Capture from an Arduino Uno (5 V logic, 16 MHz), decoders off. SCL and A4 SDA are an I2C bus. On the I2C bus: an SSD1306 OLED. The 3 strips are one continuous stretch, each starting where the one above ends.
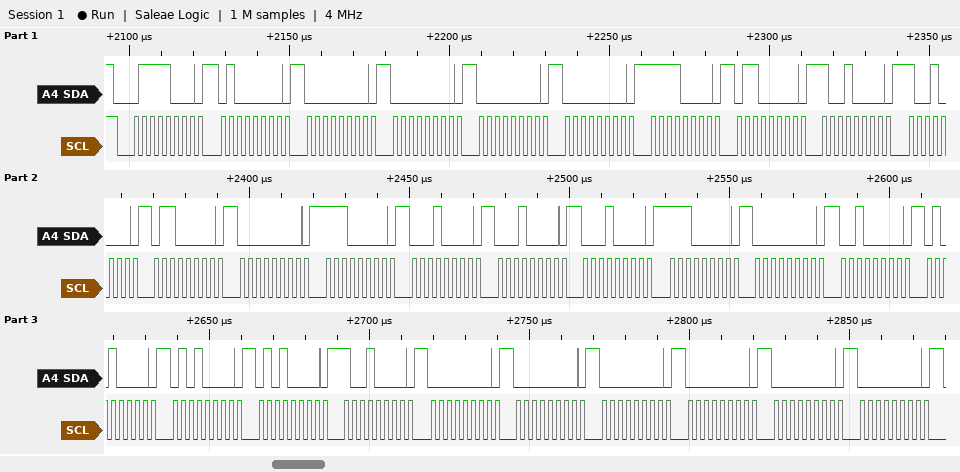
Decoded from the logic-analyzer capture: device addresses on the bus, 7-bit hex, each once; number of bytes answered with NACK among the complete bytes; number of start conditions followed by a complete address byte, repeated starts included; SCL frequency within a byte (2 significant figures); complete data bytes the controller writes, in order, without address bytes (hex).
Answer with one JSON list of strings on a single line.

["0x3C", "0", "1", "400 kHz", "40 00 00 00 00 F0 60 90 90 60 00 E0 10 10 10 E0 00 20 50 50 50 90 00 00 00 00 00 00"]
